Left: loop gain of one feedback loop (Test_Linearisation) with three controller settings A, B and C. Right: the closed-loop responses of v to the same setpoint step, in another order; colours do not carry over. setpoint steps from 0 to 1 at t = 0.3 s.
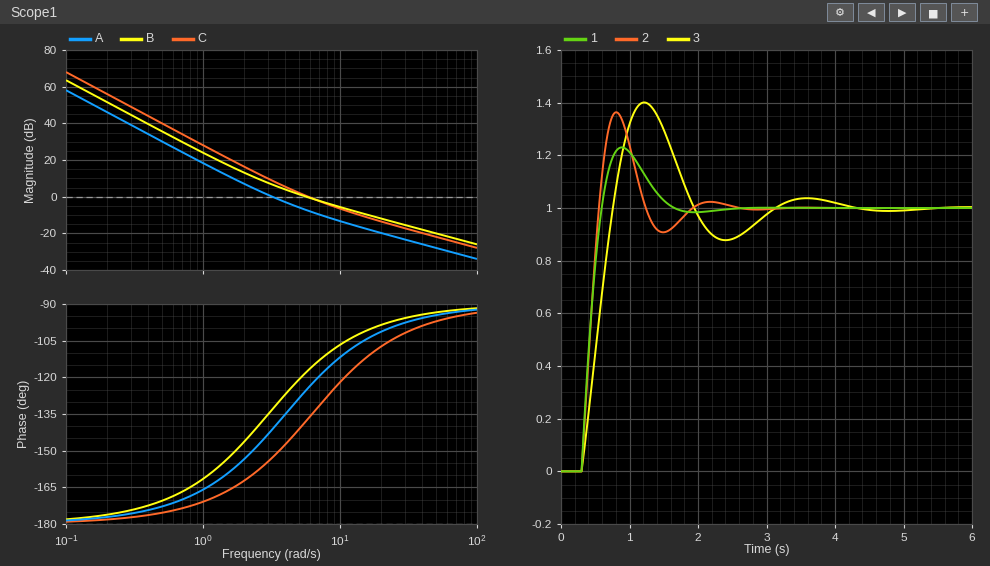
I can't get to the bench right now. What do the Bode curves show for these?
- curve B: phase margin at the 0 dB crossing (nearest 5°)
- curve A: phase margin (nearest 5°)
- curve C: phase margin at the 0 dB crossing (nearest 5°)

60°
40°
45°
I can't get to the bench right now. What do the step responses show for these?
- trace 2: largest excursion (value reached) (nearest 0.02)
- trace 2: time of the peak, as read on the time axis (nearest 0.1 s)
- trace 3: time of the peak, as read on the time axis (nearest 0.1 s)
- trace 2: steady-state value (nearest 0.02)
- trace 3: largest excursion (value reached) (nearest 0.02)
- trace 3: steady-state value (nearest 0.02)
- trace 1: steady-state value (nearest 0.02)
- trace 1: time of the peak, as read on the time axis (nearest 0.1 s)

1.36
0.8 s
1.2 s
1.00
1.40
1.00
1.00
0.9 s
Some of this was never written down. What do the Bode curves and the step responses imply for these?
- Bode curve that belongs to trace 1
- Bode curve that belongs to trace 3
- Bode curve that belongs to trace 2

B
A
C
